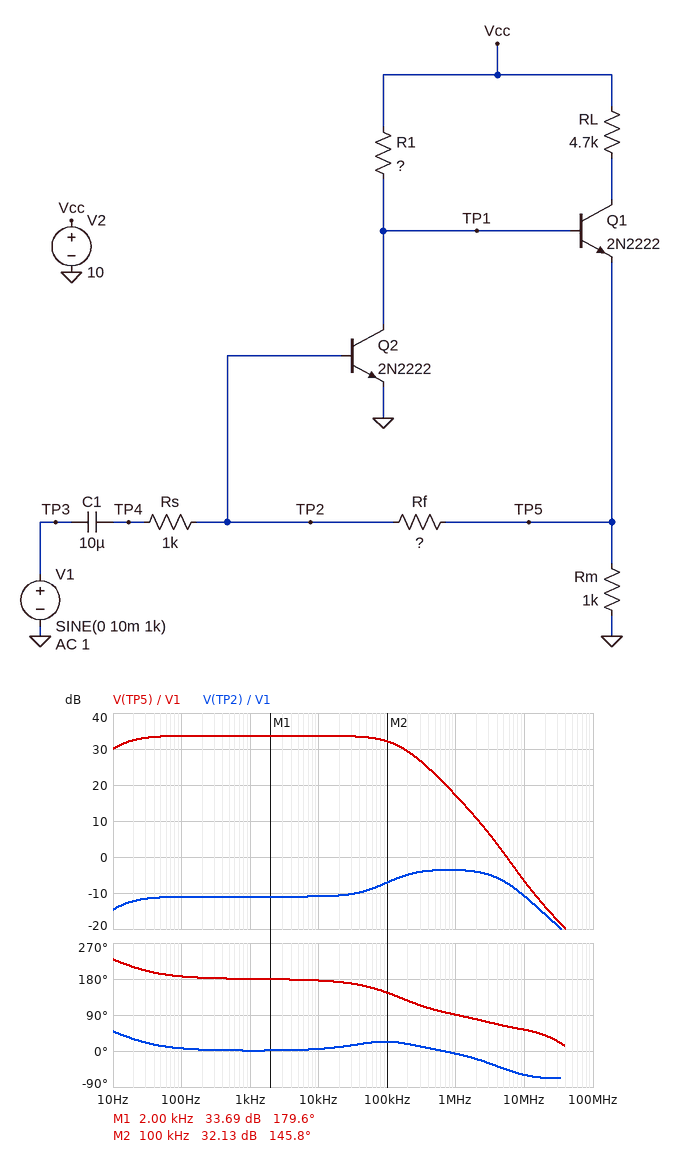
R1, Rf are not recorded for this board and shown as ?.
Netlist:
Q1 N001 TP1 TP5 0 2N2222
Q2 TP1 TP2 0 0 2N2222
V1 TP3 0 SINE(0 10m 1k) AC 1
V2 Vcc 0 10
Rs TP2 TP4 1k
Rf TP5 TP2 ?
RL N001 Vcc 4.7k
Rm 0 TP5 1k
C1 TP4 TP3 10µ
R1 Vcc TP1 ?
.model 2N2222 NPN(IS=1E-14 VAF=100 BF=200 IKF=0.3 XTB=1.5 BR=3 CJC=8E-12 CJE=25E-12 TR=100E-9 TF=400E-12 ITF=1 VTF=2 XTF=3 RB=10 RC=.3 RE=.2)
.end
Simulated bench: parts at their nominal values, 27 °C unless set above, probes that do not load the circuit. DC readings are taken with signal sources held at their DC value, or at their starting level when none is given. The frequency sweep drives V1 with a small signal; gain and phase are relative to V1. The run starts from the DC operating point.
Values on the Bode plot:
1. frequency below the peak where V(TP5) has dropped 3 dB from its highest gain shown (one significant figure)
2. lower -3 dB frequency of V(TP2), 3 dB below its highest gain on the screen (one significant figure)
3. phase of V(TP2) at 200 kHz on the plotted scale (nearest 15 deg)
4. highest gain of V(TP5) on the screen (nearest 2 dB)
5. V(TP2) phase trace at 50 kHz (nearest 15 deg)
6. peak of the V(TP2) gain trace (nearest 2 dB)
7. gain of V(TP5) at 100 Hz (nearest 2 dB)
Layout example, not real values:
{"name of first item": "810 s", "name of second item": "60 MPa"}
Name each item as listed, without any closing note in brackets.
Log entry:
{"frequency below the peak where V(TP5) has dropped 3 dB from its highest gain shown": "10 Hz", "lower -3 dB frequency of V(TP2), 3 dB below its highest gain on the screen": "100 kHz", "phase of V(TP2) at 200 kHz on the plotted scale": "15 deg", "highest gain of V(TP5) on the screen": "34 dB", "V(TP2) phase trace at 50 kHz": "15 deg", "peak of the V(TP2) gain trace": "-4 dB", "gain of V(TP5) at 100 Hz": "34 dB"}
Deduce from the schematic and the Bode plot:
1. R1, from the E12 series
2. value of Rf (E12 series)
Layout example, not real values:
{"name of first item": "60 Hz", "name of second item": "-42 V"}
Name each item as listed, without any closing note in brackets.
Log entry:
{"R1, from the E12 series": "150 kΩ", "value of Rf": "68 kΩ"}
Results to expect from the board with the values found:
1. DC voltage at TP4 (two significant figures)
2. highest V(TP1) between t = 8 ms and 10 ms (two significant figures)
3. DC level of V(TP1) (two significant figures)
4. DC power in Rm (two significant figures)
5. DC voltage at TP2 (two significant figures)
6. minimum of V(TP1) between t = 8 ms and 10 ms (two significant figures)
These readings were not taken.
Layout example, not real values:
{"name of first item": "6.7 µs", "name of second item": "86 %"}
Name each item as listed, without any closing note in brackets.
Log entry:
{"DC voltage at TP4": "580 mV", "highest V(TP1) between t = 8 ms and 10 ms": "1.7 V", "DC level of V(TP1)": "1.2 V", "DC power in Rm": "360 µW", "DC voltage at TP2": "580 mV", "minimum of V(TP1) between t = 8 ms and 10 ms": "710 mV"}
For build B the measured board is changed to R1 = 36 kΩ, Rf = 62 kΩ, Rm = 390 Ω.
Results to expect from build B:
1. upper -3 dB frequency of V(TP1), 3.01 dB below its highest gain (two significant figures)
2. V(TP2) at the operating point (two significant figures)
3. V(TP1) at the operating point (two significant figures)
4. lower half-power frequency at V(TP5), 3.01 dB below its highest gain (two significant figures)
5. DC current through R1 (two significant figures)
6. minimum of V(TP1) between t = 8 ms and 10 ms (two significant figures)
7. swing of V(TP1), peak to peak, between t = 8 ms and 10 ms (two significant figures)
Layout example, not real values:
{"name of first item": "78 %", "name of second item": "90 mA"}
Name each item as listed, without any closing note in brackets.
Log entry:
{"upper -3 dB frequency of V(TP1), 3.01 dB below its highest gain": "180 kHz", "V(TP2) at the operating point": "620 mV", "V(TP1) at the operating point": "1.4 V", "lower half-power frequency at V(TP5), 3.01 dB below its highest gain": "12 Hz", "DC current through R1": "240 µA", "minimum of V(TP1) between t = 8 ms and 10 ms": "920 mV", "swing of V(TP1), peak to peak, between t = 8 ms and 10 ms": "540 mV"}
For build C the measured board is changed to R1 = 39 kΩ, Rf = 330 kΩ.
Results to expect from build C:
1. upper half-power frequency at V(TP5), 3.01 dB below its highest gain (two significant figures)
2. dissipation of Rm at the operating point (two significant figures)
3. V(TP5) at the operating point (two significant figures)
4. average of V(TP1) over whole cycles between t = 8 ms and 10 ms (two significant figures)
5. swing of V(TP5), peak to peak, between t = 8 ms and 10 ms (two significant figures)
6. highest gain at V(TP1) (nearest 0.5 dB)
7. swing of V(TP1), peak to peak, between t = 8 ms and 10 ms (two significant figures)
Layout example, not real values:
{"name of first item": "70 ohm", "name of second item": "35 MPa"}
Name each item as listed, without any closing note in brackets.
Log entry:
{"upper half-power frequency at V(TP5), 3.01 dB below its highest gain": "110 kHz", "dissipation of Rm at the operating point": "920 µW", "V(TP5) at the operating point": "960 mV", "average of V(TP1) over whole cycles between t = 8 ms and 10 ms": "1.5 V", "swing of V(TP5), peak to peak, between t = 8 ms and 10 ms": "1.8 V", "highest gain at V(TP1)": "43.0 dB", "swing of V(TP1), peak to peak, between t = 8 ms and 10 ms": "2.3 V"}
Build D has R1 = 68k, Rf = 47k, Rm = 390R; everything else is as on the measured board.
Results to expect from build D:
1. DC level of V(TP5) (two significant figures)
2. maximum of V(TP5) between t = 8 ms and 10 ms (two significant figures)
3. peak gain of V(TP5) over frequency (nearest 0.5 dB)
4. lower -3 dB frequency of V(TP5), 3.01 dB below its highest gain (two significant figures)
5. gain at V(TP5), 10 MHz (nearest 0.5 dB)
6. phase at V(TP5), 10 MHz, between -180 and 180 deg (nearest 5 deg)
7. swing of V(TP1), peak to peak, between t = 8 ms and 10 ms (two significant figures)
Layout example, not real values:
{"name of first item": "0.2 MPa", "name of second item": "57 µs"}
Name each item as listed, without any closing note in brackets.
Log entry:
{"DC level of V(TP5)": "630 mV", "maximum of V(TP5) between t = 8 ms and 10 ms": "770 mV", "peak gain of V(TP5) over frequency": "31.0 dB", "lower -3 dB frequency of V(TP5), 3.01 dB below its highest gain": "12 Hz", "gain at V(TP5), 10 MHz": "-7.0 dB", "phase at V(TP5), 10 MHz, between -180 and 180 deg": "70 deg", "swing of V(TP1), peak to peak, between t = 8 ms and 10 ms": "500 mV"}
